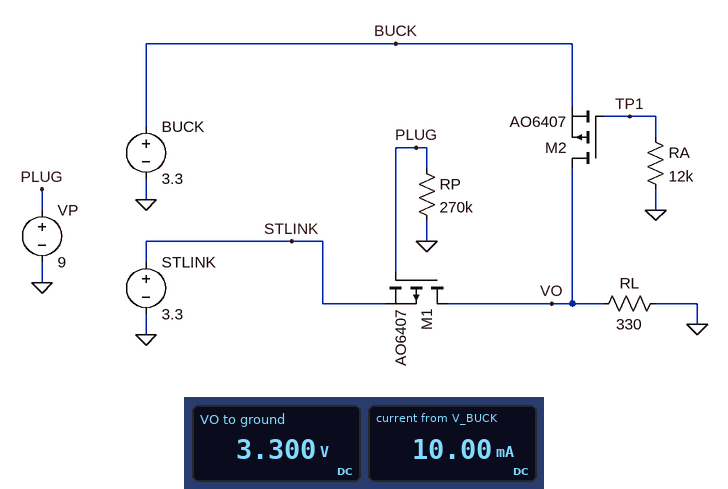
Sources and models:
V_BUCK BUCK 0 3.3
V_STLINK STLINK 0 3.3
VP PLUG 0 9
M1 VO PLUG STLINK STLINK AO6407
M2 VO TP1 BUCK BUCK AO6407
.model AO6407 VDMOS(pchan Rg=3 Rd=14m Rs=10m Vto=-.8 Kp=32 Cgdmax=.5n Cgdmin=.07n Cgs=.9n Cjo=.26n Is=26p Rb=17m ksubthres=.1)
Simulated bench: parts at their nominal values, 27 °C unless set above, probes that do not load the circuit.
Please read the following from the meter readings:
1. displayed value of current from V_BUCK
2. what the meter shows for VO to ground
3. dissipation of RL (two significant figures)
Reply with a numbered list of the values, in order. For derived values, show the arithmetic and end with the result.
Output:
1. 10.00 mA
2. 3.300 V
3. (3.3 V)^2 / 330 Ω = 33 mW
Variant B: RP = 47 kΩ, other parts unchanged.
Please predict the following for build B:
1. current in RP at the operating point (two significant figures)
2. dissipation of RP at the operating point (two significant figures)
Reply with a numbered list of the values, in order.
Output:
1. 190 µA
2. 1.7 mW
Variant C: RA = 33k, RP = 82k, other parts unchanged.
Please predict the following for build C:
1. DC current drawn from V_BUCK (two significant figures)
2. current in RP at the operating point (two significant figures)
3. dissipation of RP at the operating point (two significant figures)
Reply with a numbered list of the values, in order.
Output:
1. 10 mA
2. 110 µA
3. 990 µW
